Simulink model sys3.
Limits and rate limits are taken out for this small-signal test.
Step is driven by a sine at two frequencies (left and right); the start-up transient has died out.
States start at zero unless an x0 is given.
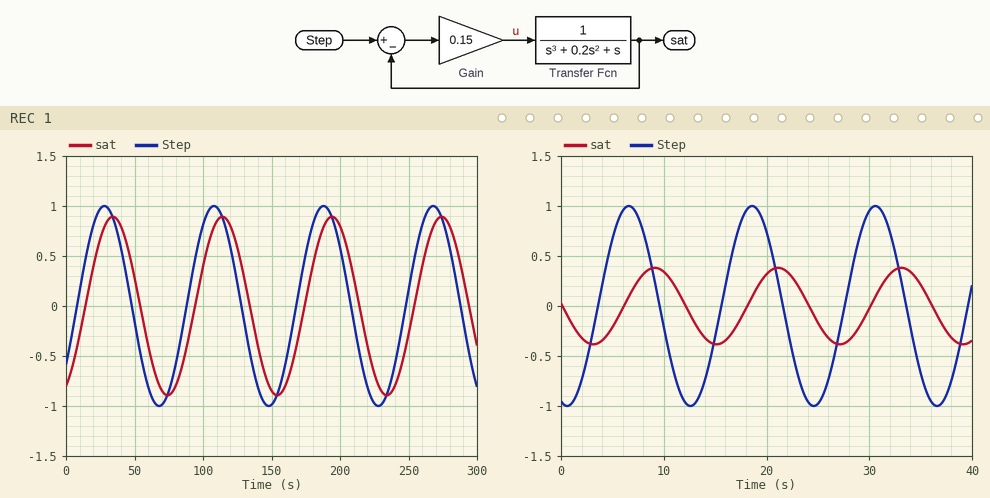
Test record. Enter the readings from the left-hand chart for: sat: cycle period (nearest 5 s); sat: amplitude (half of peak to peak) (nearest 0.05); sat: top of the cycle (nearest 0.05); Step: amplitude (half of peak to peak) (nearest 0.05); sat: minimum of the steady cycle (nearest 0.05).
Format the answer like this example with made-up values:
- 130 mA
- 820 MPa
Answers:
- 80 s
- 0.90
- 0.90
- 1.00
- -0.90
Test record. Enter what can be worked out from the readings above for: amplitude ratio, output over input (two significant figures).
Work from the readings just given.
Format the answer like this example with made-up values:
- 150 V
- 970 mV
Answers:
- 0.90
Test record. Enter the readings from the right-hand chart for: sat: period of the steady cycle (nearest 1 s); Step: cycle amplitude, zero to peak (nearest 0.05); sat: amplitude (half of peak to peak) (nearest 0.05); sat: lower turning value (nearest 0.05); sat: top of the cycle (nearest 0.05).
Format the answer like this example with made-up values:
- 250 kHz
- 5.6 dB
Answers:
- 12 s
- 1.00
- 0.40
- -0.40
- 0.40
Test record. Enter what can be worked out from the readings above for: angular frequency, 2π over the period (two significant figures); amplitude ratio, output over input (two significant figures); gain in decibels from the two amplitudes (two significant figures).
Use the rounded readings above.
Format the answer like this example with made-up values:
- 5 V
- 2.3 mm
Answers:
- 0.52 rad/s
- 0.40
- -8.0 dB
